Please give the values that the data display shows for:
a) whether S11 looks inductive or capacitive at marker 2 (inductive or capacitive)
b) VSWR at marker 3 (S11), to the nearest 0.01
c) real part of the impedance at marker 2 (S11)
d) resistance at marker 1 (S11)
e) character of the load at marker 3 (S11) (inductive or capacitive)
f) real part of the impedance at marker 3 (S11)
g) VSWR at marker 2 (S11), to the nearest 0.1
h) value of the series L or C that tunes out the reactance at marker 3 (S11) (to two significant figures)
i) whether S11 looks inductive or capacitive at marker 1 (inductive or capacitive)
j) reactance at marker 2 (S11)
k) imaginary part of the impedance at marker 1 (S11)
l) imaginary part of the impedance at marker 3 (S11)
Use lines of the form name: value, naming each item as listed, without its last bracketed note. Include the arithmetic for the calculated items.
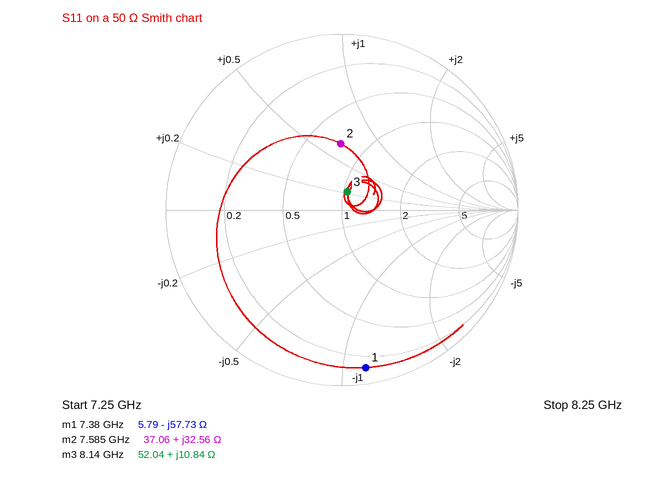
whether S11 looks inductive or capacitive at marker 2: inductive
VSWR at marker 3 (S11), to the nearest 0.01: 1.24
real part of the impedance at marker 2: 37.06 Ω
resistance at marker 1: 5.79 Ω
character of the load at marker 3 (S11): inductive
real part of the impedance at marker 3: 52.04 Ω
VSWR at marker 2 (S11), to the nearest 0.1: 2.2
value of the series L or C that tunes out the reactance at marker 3 (S11): C = 1/(2π × 8.14 GHz × 10.84 Ω) ≈ 1.8 pF
whether S11 looks inductive or capacitive at marker 1: capacitive
reactance at marker 2: +32.56 Ω
imaginary part of the impedance at marker 1: -57.73 Ω
imaginary part of the impedance at marker 3: +10.84 Ω
